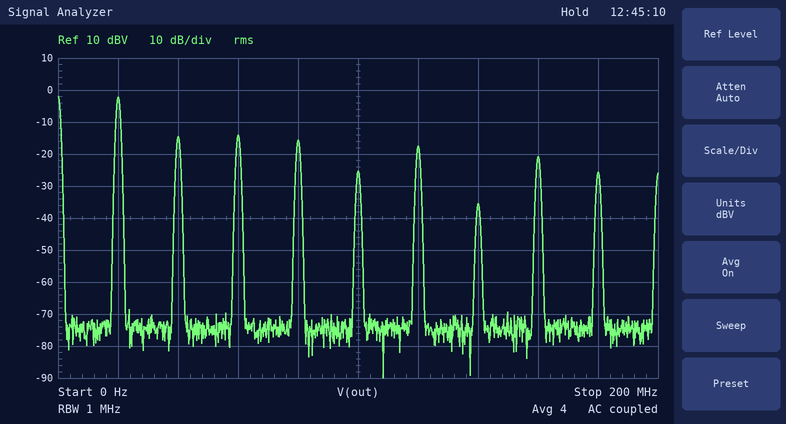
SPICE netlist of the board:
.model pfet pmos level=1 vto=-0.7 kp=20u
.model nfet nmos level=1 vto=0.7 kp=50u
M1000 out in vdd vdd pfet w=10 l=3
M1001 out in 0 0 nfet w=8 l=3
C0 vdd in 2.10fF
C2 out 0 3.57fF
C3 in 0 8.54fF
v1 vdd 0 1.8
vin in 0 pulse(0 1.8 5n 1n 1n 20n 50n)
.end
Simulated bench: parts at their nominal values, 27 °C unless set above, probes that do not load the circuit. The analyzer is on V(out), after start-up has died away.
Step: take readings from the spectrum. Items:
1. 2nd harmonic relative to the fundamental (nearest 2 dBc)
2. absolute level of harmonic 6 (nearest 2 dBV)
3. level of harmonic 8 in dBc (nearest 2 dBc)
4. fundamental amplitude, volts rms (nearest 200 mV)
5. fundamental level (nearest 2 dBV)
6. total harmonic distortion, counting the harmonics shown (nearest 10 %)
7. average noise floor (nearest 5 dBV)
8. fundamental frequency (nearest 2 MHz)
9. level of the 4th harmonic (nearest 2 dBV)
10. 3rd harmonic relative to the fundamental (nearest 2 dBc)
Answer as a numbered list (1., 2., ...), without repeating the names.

1. -12 dBc
2. -18 dBV
3. -18 dBc
4. 800 mV
5. -2 dBV
6. 50 %
7. -75 dBV
8. 20 MHz
9. -16 dBV
10. -12 dBc
